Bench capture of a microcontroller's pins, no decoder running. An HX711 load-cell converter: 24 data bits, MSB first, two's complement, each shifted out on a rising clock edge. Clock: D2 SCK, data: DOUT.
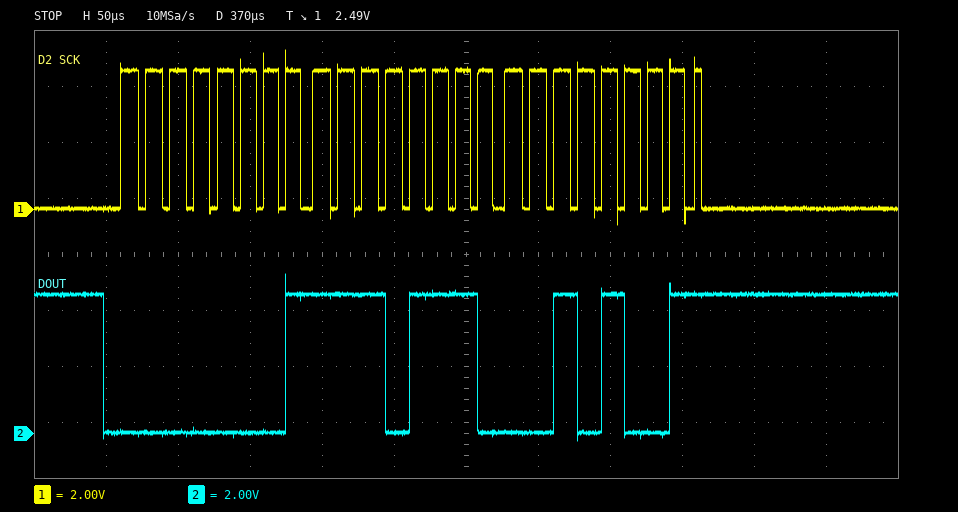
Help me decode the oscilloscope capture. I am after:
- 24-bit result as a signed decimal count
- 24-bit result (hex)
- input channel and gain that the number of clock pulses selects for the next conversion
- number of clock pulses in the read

126505
0x01EE29
channel A, gain 128
25
